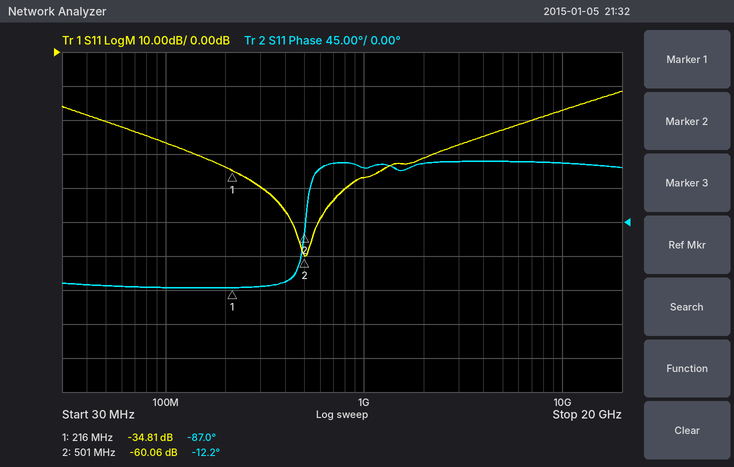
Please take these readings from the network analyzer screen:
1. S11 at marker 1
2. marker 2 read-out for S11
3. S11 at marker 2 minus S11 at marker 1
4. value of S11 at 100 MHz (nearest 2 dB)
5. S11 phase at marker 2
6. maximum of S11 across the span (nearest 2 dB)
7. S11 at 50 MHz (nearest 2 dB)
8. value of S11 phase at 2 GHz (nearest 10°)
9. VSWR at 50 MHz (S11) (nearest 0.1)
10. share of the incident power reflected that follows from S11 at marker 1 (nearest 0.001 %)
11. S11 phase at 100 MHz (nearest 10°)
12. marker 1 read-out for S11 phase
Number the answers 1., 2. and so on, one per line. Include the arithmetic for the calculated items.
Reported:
1. -34.81 dB
2. -60.06 dB
3. -60.06 − (-34.81) = -25.25 dB
4. -26 dB
5. -12.2°
6. -12 dB
7. -20 dB
8. 80°
9. |Γ| = 10^(-20/20) = 0.1000; VSWR = (1 + 0.1000)/(1 − 0.1000) ≈ 1.2
10. 10^(-34.81/10) ≈ 0.033 %
11. -90°
12. -87.0°
